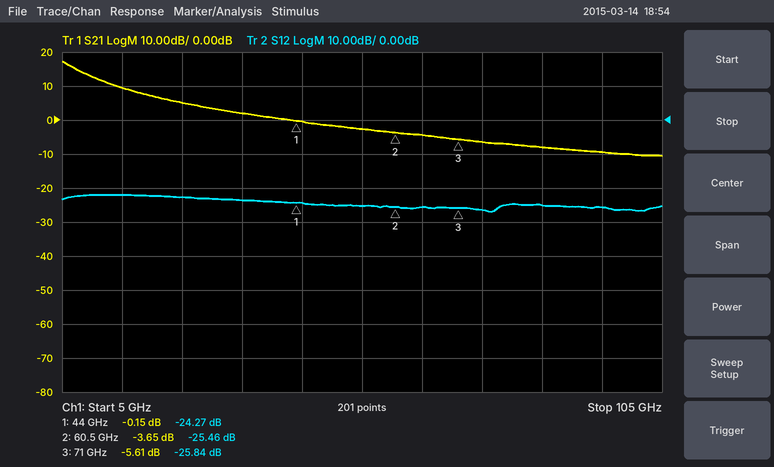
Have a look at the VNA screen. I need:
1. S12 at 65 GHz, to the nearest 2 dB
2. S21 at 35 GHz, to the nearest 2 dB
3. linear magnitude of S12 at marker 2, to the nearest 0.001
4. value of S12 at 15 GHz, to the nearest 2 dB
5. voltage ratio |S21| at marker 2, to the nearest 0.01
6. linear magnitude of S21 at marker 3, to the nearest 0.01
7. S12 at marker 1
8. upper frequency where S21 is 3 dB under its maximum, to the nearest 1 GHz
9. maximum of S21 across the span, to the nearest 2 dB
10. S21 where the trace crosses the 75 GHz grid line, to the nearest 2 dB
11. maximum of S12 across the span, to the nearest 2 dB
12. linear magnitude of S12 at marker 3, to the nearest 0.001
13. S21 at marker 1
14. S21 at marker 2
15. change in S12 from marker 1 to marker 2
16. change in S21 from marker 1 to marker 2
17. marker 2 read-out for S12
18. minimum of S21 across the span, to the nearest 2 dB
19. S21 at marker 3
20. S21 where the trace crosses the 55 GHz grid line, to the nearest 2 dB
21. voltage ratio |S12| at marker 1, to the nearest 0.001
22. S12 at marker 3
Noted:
-26 dB
2 dB
0.053
-22 dB
0.66
0.52
-24.27 dB
8 GHz
18 dB
-6 dB
-22 dB
0.051
-0.15 dB
-3.65 dB
-1.19 dB
-3.50 dB
-25.46 dB
-10 dB
-5.61 dB
-2 dB
0.061
-25.84 dB
